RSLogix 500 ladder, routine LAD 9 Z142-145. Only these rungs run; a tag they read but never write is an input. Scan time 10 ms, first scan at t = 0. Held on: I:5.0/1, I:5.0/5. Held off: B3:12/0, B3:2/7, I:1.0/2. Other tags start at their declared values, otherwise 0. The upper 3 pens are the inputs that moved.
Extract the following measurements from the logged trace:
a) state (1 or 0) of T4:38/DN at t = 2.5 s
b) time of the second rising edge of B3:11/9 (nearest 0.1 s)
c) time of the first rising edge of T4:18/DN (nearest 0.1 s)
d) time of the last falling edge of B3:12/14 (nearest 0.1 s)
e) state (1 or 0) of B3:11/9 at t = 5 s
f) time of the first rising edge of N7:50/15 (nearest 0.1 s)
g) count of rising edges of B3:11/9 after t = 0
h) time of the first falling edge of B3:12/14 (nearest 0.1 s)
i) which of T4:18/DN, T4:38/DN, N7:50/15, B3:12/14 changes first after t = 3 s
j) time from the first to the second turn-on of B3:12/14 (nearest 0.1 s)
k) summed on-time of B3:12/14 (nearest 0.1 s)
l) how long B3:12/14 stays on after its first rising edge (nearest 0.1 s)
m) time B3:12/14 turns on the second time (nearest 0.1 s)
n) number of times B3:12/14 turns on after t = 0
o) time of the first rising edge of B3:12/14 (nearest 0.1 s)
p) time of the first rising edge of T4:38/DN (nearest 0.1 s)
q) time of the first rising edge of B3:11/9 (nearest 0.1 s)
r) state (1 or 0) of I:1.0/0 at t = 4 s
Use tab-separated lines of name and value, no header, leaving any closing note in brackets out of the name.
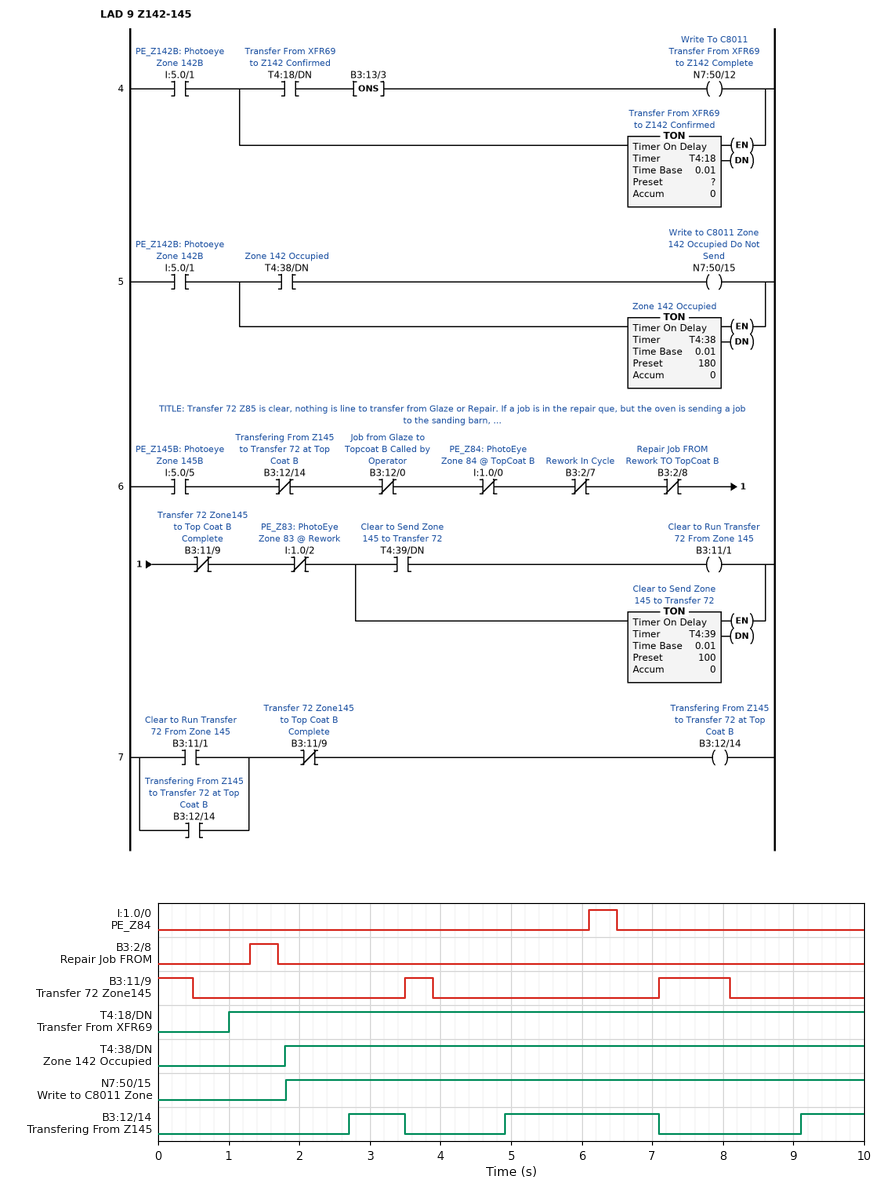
state (1 or 0) of T4:38/DN at t = 2.5 s	1
time of the second rising edge of B3:11/9	7.1 s
time of the first rising edge of T4:18/DN	1.0 s
time of the last falling edge of B3:12/14	7.1 s
state (1 or 0) of B3:11/9 at t = 5 s	0
time of the first rising edge of N7:50/15	1.8 s
count of rising edges of B3:11/9 after t = 0	2
time of the first falling edge of B3:12/14	3.5 s
which of T4:18/DN, T4:38/DN, N7:50/15, B3:12/14 changes first after t = 3 s	B3:12/14
time from the first to the second turn-on of B3:12/14	2.2 s
summed on-time of B3:12/14	3.9 s
how long B3:12/14 stays on after its first rising edge	0.8 s
time B3:12/14 turns on the second time	4.9 s
number of times B3:12/14 turns on after t = 0	3
time of the first rising edge of B3:12/14	2.7 s
time of the first rising edge of T4:38/DN	1.8 s
time of the first rising edge of B3:11/9	3.5 s
state (1 or 0) of I:1.0/0 at t = 4 s	0
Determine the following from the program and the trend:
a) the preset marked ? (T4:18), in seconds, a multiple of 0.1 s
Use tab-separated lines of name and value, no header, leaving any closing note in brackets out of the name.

the preset marked ? (T4:18), in seconds, a multiple of 0.1 s	1.0 s
